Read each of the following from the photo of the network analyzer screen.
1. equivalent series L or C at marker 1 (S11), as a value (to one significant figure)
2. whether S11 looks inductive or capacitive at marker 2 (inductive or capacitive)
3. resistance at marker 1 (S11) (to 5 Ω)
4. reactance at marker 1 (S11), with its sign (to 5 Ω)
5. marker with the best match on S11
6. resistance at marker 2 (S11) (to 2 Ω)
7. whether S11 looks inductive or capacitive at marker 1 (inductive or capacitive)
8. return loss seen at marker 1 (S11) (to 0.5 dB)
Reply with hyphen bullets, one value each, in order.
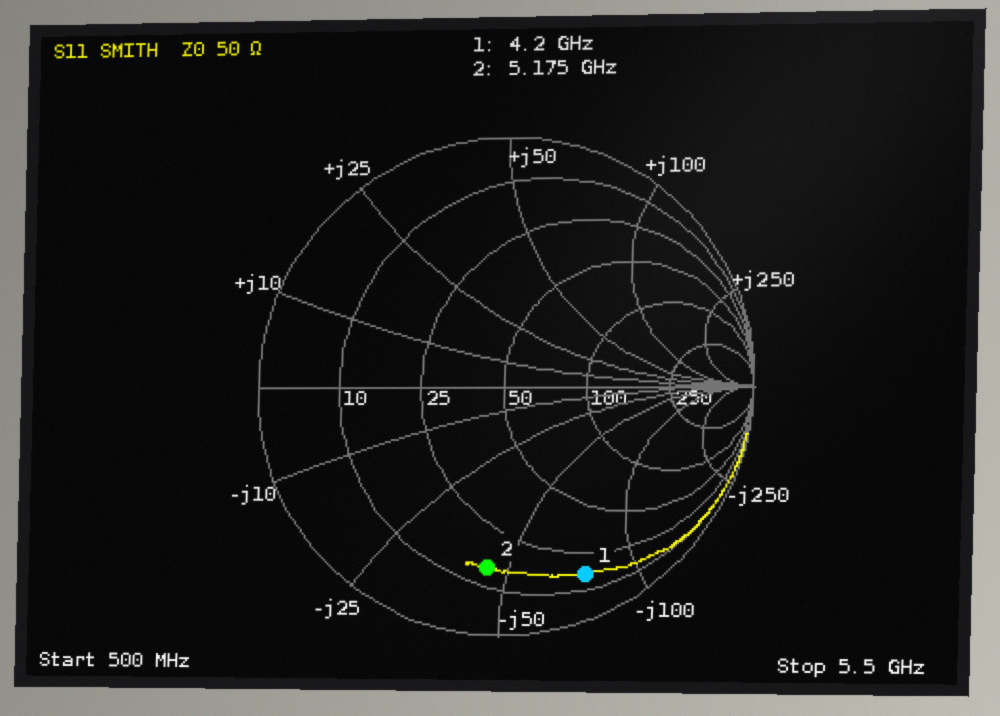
- 500 fF
- capacitive
- 15 Ω
- -75 Ω
- marker 2
- 14 Ω
- capacitive
- 1.5 dB
